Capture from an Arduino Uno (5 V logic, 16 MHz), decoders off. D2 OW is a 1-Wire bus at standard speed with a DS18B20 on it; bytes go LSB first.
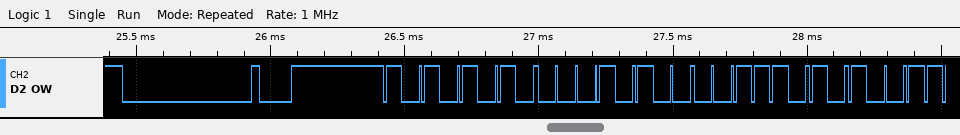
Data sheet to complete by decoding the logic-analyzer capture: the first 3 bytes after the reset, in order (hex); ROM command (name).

55 28 5C
Match ROM
